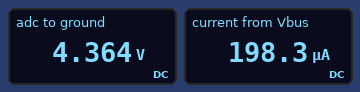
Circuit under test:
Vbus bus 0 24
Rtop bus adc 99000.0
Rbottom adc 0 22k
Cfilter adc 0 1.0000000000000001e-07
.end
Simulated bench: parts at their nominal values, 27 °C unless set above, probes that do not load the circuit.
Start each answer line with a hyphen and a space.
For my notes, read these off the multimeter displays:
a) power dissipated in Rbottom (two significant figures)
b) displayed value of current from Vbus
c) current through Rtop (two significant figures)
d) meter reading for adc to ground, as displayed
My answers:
- 870 µW
- 198.3 µA
- 200 µA
- 4.364 V
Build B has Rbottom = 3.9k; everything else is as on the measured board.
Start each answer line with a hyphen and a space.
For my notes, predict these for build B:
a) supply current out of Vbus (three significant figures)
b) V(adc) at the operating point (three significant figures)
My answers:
- 233 µA
- 910 mV
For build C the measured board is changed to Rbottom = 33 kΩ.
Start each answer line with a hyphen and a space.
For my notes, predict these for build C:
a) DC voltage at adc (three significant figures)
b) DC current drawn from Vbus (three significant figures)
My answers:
- 6.00 V
- 182 µA
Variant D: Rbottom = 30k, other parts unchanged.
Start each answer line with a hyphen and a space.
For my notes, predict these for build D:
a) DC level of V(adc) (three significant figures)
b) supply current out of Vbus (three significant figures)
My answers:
- 5.58 V
- 186 µA
